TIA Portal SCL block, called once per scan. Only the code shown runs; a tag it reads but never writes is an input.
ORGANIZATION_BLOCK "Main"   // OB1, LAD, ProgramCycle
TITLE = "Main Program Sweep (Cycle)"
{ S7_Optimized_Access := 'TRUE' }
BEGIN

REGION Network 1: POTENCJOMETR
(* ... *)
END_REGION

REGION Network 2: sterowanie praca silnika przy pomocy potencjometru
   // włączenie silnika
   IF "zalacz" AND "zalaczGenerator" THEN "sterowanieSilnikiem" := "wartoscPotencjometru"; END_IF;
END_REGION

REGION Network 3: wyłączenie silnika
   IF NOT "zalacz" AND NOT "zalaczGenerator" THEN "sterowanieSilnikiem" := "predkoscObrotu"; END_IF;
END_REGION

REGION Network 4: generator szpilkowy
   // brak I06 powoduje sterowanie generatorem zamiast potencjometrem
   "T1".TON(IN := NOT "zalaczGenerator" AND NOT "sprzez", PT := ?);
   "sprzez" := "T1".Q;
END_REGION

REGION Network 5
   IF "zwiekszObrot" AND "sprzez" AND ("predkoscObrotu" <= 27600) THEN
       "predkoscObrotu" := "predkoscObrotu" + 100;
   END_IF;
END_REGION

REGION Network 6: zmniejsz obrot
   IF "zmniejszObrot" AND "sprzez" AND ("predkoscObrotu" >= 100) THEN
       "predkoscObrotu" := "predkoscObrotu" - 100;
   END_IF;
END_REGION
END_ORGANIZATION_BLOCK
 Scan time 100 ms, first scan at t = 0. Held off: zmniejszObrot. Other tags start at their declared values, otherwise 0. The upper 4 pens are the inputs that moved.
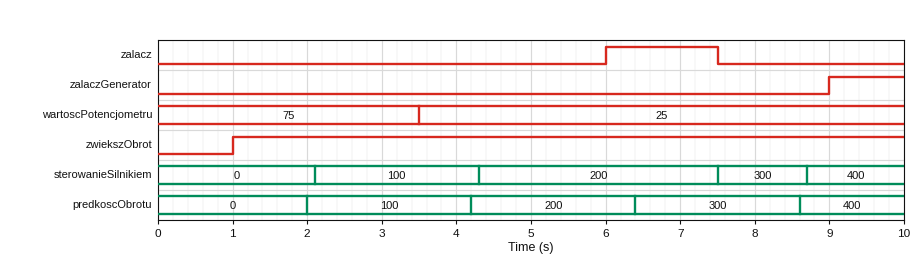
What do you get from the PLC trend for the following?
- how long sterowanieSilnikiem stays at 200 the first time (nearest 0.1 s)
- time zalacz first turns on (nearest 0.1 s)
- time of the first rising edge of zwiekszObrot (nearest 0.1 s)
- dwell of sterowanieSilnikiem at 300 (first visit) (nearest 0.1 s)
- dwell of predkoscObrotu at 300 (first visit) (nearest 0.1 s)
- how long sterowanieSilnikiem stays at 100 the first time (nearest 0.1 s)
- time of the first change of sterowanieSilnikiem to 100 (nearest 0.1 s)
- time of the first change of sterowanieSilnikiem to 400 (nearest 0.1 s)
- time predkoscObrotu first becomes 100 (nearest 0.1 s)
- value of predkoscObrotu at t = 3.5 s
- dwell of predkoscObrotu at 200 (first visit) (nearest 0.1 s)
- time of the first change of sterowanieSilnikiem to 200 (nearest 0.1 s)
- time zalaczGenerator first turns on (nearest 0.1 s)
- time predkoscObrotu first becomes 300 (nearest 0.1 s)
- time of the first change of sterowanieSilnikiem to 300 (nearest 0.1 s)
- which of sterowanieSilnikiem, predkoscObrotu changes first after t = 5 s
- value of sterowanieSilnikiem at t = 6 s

3.2 s
6.0 s
1.0 s
1.2 s
2.2 s
2.2 s
2.1 s
8.7 s
2.0 s
100
2.2 s
4.3 s
9.0 s
6.4 s
7.5 s
predkoscObrotu
200
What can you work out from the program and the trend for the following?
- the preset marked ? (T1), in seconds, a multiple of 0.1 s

2.0 s
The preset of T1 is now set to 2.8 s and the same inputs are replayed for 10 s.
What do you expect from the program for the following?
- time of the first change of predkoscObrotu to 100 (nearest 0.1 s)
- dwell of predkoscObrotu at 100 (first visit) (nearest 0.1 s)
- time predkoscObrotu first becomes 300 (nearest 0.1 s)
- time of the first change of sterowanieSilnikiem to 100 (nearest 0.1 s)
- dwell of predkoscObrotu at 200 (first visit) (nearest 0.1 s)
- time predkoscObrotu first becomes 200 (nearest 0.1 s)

2.8 s
3.0 s
8.8 s
2.9 s
3.0 s
5.8 s
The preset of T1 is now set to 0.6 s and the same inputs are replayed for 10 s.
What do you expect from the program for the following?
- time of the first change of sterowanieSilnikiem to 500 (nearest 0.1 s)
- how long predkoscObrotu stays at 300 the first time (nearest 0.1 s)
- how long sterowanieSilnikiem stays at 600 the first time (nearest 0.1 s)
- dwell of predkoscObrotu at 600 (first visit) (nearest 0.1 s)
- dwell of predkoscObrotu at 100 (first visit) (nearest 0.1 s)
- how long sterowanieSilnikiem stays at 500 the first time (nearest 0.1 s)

4.7 s
0.8 s
2.0 s
0.8 s
0.8 s
0.8 s
